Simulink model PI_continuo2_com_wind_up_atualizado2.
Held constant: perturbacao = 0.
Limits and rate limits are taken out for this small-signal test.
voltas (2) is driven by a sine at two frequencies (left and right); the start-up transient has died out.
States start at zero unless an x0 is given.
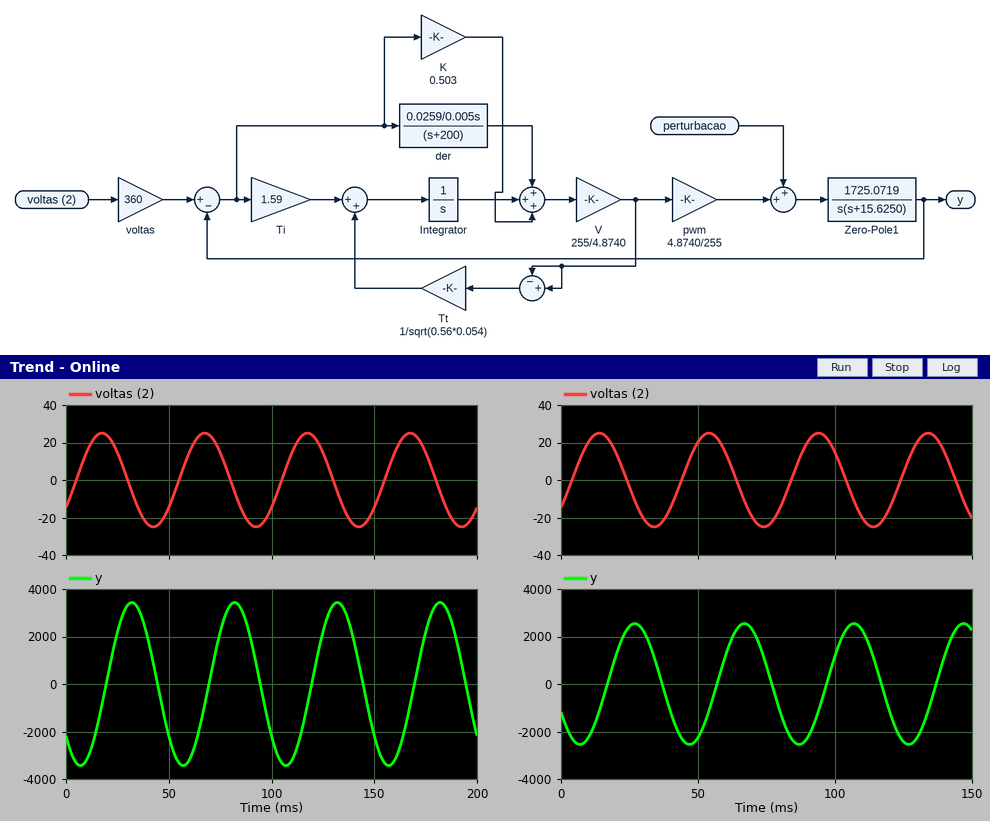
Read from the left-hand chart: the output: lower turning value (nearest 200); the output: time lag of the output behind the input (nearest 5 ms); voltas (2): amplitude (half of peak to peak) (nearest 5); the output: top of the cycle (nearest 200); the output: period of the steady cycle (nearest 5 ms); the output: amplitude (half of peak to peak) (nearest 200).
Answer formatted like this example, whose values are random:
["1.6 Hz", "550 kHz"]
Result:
["-3400", "15 ms", "25", "3400", "50 ms", "3400"]
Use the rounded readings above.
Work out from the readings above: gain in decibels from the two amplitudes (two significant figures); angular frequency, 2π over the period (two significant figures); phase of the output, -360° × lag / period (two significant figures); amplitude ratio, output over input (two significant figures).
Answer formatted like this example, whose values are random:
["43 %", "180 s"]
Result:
["43 dB", "0.13 rad/ms", "-110°", "140"]
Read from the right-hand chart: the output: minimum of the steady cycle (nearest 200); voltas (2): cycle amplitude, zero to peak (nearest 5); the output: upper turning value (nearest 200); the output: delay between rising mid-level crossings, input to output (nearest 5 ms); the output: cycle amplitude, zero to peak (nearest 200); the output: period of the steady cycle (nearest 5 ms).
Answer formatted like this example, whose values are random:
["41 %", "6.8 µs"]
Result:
["-2600", "25", "2600", "15 ms", "2600", "40 ms"]
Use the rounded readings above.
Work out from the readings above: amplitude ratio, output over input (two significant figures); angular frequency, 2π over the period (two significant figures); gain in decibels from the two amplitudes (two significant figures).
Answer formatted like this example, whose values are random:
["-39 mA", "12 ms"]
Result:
["100", "0.16 rad/ms", "40 dB"]
